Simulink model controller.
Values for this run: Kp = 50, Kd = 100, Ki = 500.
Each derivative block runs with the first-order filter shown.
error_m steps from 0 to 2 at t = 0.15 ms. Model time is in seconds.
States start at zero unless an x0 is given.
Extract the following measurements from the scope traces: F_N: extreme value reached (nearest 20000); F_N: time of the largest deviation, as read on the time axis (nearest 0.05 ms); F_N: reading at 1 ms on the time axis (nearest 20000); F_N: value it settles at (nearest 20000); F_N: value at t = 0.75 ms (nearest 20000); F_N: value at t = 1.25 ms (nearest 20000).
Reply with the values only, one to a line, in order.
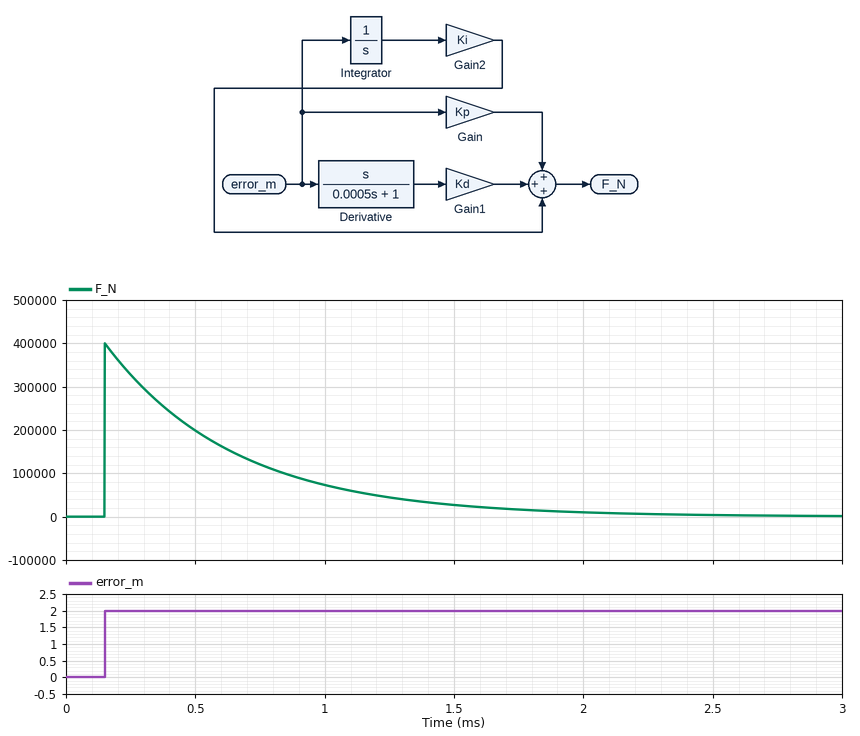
400000
0.15 ms
80000
0
120000
40000
